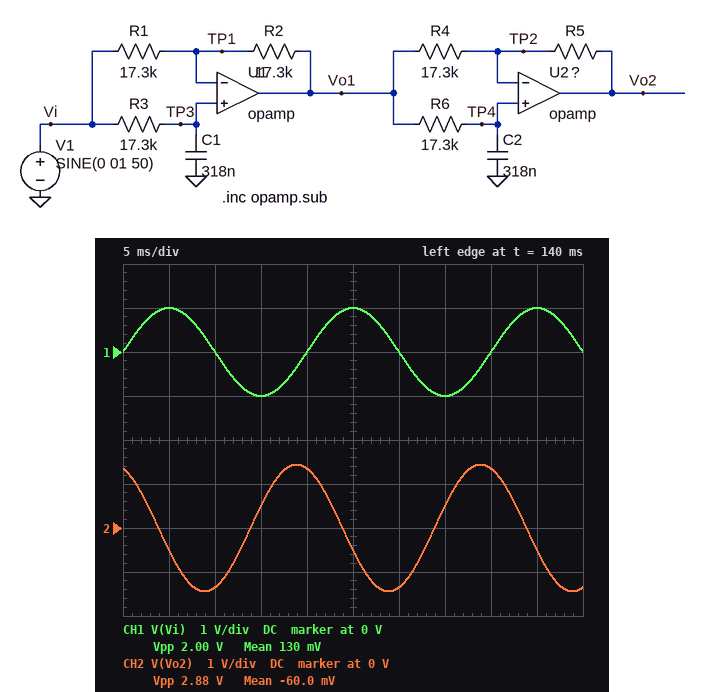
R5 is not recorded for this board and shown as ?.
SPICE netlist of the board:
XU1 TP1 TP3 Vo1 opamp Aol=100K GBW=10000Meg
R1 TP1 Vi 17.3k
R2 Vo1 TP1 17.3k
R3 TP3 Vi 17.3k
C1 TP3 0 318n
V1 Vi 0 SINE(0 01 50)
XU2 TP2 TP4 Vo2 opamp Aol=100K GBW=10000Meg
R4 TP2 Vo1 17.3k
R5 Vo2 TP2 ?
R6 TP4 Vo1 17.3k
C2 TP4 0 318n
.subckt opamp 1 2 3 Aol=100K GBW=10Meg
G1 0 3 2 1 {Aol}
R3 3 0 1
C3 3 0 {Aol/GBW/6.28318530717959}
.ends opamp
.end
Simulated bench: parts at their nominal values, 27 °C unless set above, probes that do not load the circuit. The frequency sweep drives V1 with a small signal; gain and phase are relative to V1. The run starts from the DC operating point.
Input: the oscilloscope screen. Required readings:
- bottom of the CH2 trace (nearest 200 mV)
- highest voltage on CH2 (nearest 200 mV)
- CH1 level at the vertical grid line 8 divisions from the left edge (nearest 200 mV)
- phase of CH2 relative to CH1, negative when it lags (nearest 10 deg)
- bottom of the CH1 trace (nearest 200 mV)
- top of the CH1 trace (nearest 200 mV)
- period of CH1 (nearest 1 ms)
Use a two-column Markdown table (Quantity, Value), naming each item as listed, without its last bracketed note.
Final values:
| Quantity | Value |
|---|---|
| bottom of the CH2 trace | -1.4 V |
| highest voltage on CH2 | 1.4 V |
| CH1 level at the vertical grid line 8 divisions from the left edge | 0 V |
| phase of CH2 relative to CH1, negative when it lags | 110 deg |
| bottom of the CH1 trace | -1.0 V |
| top of the CH1 trace | 1.0 V |
| period of CH1 | 20 ms |
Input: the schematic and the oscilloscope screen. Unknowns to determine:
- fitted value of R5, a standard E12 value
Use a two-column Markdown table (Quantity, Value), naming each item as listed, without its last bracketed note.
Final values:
| Quantity | Value |
|---|---|
| fitted value of R5, a standard E12 value | 27 kΩ |
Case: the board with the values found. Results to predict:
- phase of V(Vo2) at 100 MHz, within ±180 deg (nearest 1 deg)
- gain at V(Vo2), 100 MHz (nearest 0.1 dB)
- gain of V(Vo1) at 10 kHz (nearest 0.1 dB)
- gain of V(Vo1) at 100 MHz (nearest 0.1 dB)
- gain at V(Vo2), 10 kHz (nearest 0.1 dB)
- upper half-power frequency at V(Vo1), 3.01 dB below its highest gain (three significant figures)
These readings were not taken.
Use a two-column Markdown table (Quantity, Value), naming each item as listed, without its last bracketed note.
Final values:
| Quantity | Value |
|---|---|
| phase of V(Vo2) at 100 MHz, within ±180 deg | -3 deg |
| gain at V(Vo2), 100 MHz | 3.9 dB |
| gain of V(Vo1) at 10 kHz | 0 dB |
| gain of V(Vo1) at 100 MHz | 0 dB |
| gain at V(Vo2), 10 kHz | 3.9 dB |
| upper half-power frequency at V(Vo1), 3.01 dB below its highest gain | 5.00 GHz |
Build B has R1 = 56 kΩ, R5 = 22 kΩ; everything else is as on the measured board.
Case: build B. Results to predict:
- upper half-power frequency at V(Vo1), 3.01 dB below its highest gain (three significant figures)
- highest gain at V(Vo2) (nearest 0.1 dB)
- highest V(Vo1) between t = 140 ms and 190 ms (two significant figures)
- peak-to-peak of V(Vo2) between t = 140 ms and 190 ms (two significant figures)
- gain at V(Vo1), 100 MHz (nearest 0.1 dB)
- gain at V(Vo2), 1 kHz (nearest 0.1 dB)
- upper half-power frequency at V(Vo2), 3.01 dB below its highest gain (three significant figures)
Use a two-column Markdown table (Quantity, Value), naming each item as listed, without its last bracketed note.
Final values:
| Quantity | Value |
|---|---|
| upper half-power frequency at V(Vo1), 3.01 dB below its highest gain | 32.2 Hz |
| highest gain at V(Vo2) | 0 dB |
| highest V(Vo1) between t = 140 ms and 190 ms | 570 mV |
| peak-to-peak of V(Vo2) between t = 140 ms and 190 ms | 1.4 V |
| gain at V(Vo1), 100 MHz | -10.2 dB |
| gain at V(Vo2), 1 kHz | -8.1 dB |
| upper half-power frequency at V(Vo2), 3.01 dB below its highest gain | 46.8 Hz |
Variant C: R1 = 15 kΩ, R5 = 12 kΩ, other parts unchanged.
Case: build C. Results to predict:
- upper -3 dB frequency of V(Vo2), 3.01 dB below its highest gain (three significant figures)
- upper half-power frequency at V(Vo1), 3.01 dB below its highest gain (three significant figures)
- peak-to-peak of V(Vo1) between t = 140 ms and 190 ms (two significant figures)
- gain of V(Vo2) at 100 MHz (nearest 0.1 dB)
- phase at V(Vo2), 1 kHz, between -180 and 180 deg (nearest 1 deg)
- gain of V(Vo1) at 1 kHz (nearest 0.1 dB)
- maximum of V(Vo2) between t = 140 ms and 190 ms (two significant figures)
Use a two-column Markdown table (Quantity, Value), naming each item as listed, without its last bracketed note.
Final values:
| Quantity | Value |
|---|---|
| upper -3 dB frequency of V(Vo2), 3.01 dB below its highest gain | 1.87 GHz |
| upper half-power frequency at V(Vo1), 3.01 dB below its highest gain | 4.64 GHz |
| peak-to-peak of V(Vo1) between t = 140 ms and 190 ms | 2.2 V |
| gain of V(Vo2) at 100 MHz | -1.9 dB |
| phase at V(Vo2), 1 kHz, between -180 and 180 deg | 7 deg |
| gain of V(Vo1) at 1 kHz | 1.2 dB |
| maximum of V(Vo2) between t = 140 ms and 190 ms | 870 mV |
